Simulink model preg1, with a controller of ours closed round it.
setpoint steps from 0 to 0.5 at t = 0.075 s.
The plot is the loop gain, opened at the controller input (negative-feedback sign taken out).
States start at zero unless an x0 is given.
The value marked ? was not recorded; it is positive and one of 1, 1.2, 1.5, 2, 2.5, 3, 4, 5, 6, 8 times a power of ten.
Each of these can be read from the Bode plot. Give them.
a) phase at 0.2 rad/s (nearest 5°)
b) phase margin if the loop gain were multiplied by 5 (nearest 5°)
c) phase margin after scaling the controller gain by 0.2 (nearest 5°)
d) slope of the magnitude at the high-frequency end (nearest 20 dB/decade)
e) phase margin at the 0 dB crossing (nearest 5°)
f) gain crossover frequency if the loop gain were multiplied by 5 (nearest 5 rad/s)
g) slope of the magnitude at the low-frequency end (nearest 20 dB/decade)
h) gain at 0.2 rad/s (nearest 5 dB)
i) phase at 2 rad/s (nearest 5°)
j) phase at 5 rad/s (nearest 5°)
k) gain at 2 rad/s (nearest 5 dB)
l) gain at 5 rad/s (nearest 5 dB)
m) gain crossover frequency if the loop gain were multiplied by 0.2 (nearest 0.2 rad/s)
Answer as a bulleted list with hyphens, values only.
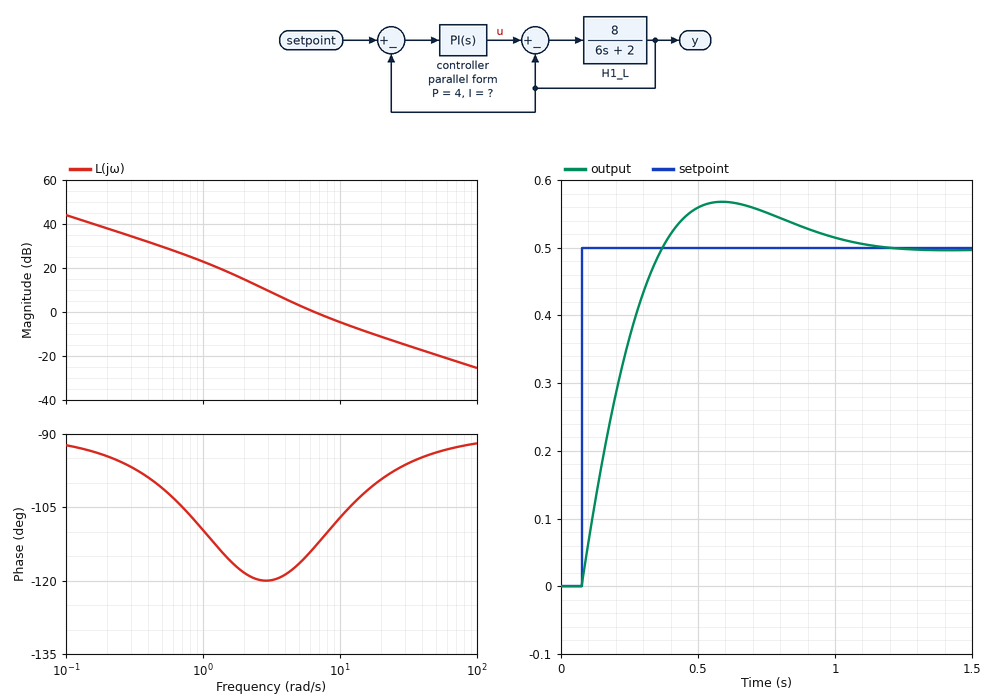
- -95°
- 85°
- 60°
- -20 dB/decade
- 65°
- 25 rad/s
- -20 dB/decade
- 40 dB
- -120°
- -115°
- 15 dB
- 5 dB
- 2.2 rad/s
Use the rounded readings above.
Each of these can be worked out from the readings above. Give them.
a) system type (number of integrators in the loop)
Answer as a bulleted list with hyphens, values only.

- 1
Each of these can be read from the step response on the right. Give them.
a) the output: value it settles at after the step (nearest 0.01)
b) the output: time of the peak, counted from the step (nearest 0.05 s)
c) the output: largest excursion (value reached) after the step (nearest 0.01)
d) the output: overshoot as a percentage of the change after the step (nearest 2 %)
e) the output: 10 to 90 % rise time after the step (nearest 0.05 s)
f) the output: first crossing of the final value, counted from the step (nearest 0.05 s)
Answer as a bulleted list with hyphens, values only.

- 0.50
- 0.50 s
- 0.57
- 14 %
- 0.20 s
- 0.30 s
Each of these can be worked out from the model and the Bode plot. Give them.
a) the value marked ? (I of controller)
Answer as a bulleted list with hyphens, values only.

- 20
